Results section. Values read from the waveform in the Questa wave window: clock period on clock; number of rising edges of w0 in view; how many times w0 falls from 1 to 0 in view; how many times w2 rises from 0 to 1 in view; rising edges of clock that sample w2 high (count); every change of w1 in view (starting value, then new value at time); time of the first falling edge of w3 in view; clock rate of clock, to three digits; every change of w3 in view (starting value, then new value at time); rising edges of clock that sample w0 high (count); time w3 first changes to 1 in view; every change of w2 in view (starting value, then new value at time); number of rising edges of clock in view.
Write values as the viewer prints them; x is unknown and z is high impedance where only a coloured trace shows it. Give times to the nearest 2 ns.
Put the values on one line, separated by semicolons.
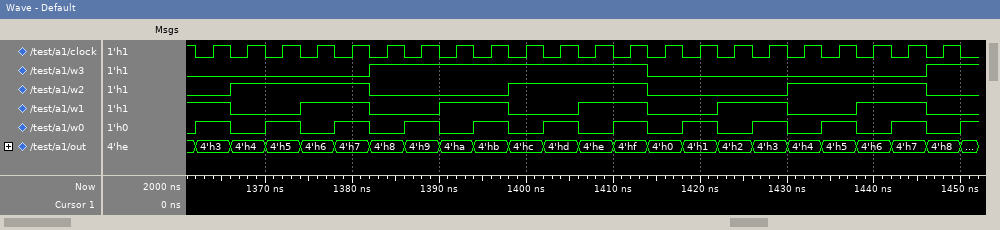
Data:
4 ns; 12; 11; 3; 12; 1, 0 at 1366 ns, 1 at 1374 ns, 0 at 1382 ns, 1 at 1390 ns, 0 at 1398 ns, 1 at 1406 ns, 0 at 1414 ns, 1 at 1422 ns, 0 at 1430 ns, 1 at 1438 ns, 0 at 1446 ns; 1414 ns; 250 MHz; 0, 1 at 1382 ns, 0 at 1414 ns, 1 at 1446 ns; 11; 1382 ns; 0, 1 at 1366 ns, 0 at 1382 ns, 1 at 1398 ns, 0 at 1414 ns, 1 at 1430 ns, 0 at 1446 ns; 22
